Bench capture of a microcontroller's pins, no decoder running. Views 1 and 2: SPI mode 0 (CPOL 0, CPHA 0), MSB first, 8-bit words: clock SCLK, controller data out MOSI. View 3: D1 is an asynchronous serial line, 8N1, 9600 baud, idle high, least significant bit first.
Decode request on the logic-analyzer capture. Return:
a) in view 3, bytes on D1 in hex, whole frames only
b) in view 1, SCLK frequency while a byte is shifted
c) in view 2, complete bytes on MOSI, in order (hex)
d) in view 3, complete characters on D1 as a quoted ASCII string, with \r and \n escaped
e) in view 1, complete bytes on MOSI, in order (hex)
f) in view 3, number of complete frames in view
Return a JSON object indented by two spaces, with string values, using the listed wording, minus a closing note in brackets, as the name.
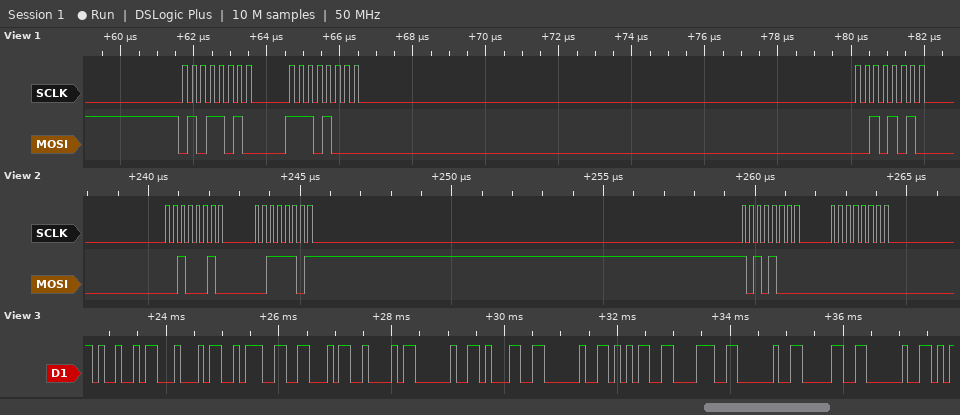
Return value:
{
  "in view 3, bytes on D1 in hex, whole frames only": "0x49 0x44 0x3A 0x46 0x42 0x20 0x31 0x20 0x35 0x38 0x20 0x30 0x20",
  "in view 1, SCLK frequency while a byte is shifted": "4 MHz",
  "in view 2, complete bytes on MOSI, in order": "22 3D A8 00",
  "in view 3, complete characters on D1 as a quoted ASCII string, with \\r and \\n escaped": "\"ID:FB 1 58 0 \"",
  "in view 1, complete bytes on MOSI, in order": "5A E8 2A",
  "in view 3, number of complete frames in view": "13"
}
